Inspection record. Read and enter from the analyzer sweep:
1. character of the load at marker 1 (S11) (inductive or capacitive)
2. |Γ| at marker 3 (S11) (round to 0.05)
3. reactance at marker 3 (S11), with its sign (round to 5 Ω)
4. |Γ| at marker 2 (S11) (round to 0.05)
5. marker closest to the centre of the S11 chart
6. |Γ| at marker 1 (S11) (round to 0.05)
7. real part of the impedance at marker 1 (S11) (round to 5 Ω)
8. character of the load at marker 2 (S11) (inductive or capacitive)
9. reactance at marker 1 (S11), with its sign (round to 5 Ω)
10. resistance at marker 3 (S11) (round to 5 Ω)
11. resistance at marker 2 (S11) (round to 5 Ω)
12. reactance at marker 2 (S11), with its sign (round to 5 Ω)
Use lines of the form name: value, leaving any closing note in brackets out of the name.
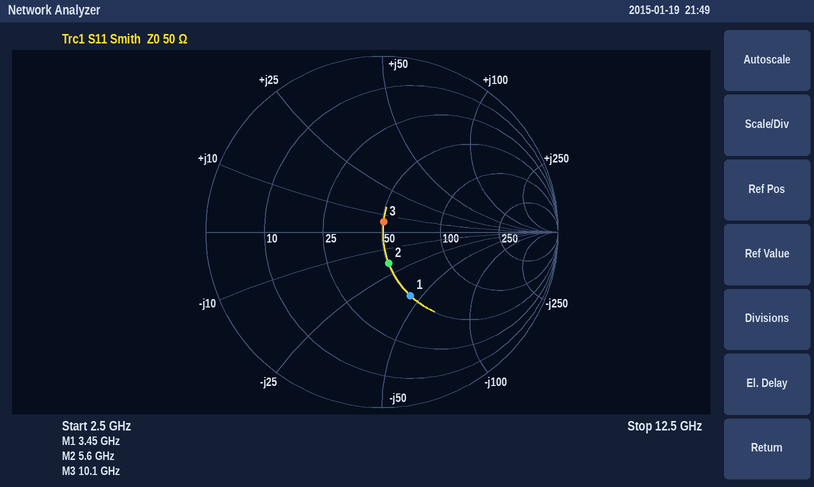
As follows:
character of the load at marker 1 (S11): capacitive
|Γ| at marker 3 (S11): 0.05
reactance at marker 3 (S11), with its sign: +5 Ω
|Γ| at marker 2 (S11): 0.20
marker closest to the centre of the S11 chart: marker 3
|Γ| at marker 1 (S11): 0.40
real part of the impedance at marker 1 (S11): 50 Ω
character of the load at marker 2 (S11): capacitive
reactance at marker 1 (S11), with its sign: -45 Ω
resistance at marker 3 (S11): 50 Ω
resistance at marker 2 (S11): 50 Ω
reactance at marker 2 (S11), with its sign: -20 Ω
